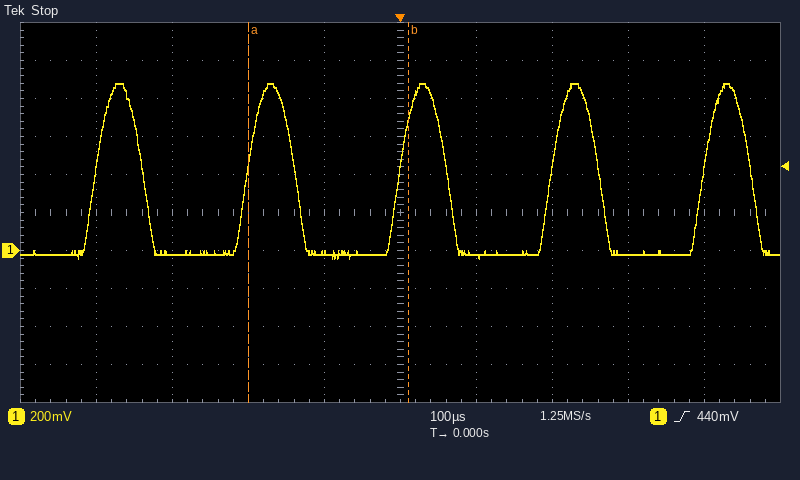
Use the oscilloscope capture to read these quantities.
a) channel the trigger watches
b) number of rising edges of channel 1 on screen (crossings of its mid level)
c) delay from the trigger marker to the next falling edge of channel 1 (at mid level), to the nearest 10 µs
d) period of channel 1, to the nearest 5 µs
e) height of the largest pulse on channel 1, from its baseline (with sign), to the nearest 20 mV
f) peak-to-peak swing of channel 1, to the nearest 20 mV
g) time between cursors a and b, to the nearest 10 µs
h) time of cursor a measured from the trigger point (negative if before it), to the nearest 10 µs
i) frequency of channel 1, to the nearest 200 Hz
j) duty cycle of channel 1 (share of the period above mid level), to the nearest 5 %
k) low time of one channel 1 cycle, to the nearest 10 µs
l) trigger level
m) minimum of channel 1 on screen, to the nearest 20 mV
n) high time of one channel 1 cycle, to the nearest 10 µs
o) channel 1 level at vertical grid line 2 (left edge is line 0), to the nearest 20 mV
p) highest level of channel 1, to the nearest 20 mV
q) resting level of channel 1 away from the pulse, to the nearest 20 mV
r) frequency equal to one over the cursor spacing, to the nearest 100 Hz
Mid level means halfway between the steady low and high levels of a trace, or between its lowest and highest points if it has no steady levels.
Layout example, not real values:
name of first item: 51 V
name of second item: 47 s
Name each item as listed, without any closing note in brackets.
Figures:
channel the trigger watches: channel 1
number of rising edges of channel 1 on screen: 5
delay from the trigger marker to the next falling edge of channel 1 (at mid level), to the nearest 10 µs: 60 µs
period of channel 1, to the nearest 5 µs: 200 µs
height of the largest pulse on channel 1, from its baseline (with sign), to the nearest 20 mV: +900 mV
peak-to-peak swing of channel 1, to the nearest 20 mV: 920 mV
time between cursors a and b, to the nearest 10 µs: 210 µs
time of cursor a measured from the trigger point (negative if before it), to the nearest 10 µs: -200 µs
frequency of channel 1, to the nearest 200 Hz: 5.0 kHz
duty cycle of channel 1 (share of the period above mid level), to the nearest 5 %: 30 %
low time of one channel 1 cycle, to the nearest 10 µs: 140 µs
trigger level: 440 mV
minimum of channel 1 on screen, to the nearest 20 mV: -40 mV
high time of one channel 1 cycle, to the nearest 10 µs: 60 µs
channel 1 level at vertical grid line 2 (left edge is line 0), to the nearest 20 mV: -20 mV
highest level of channel 1, to the nearest 20 mV: 880 mV
resting level of channel 1 away from the pulse, to the nearest 20 mV: -20 mV
frequency equal to one over the cursor spacing, to the nearest 100 Hz: 4.8 kHz
